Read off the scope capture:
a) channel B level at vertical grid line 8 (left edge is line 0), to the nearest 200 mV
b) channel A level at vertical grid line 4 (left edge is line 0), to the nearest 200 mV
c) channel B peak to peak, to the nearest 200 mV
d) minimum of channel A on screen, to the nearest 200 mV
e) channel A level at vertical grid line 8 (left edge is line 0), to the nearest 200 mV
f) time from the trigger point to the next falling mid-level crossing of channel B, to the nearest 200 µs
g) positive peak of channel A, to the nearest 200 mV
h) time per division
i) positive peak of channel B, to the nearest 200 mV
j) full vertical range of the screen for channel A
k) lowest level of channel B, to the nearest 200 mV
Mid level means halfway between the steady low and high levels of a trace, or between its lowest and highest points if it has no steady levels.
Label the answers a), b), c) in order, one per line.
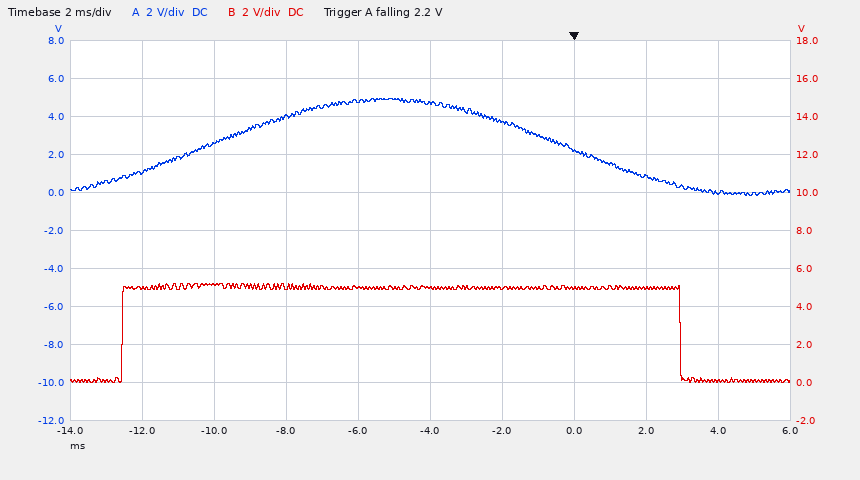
a) 5.0 V
b) 4.8 V
c) 5.2 V
d) -200 mV
e) 800 mV
f) 3.0 ms
g) 5.0 V
h) 2 ms
i) 5.2 V
j) 20 V
k) 0.0 V
